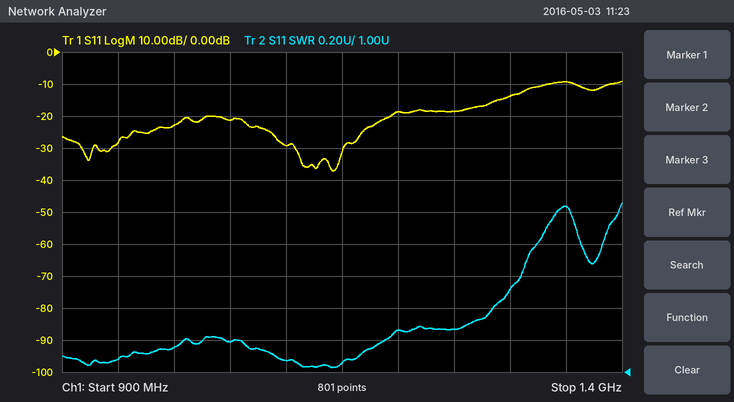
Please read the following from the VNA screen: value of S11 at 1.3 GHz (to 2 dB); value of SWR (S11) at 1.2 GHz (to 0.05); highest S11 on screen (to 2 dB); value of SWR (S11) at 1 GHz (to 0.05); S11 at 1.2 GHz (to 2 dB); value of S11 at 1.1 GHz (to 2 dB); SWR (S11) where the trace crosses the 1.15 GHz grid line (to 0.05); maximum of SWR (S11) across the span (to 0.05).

-14 dB
1.25
-10 dB
1.15
-18 dB
-30 dB
1.05
2.05
